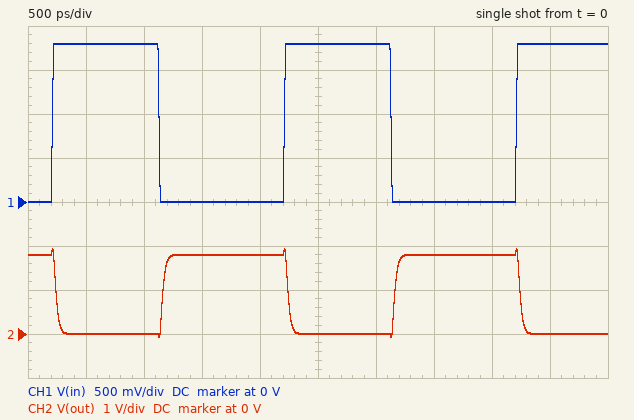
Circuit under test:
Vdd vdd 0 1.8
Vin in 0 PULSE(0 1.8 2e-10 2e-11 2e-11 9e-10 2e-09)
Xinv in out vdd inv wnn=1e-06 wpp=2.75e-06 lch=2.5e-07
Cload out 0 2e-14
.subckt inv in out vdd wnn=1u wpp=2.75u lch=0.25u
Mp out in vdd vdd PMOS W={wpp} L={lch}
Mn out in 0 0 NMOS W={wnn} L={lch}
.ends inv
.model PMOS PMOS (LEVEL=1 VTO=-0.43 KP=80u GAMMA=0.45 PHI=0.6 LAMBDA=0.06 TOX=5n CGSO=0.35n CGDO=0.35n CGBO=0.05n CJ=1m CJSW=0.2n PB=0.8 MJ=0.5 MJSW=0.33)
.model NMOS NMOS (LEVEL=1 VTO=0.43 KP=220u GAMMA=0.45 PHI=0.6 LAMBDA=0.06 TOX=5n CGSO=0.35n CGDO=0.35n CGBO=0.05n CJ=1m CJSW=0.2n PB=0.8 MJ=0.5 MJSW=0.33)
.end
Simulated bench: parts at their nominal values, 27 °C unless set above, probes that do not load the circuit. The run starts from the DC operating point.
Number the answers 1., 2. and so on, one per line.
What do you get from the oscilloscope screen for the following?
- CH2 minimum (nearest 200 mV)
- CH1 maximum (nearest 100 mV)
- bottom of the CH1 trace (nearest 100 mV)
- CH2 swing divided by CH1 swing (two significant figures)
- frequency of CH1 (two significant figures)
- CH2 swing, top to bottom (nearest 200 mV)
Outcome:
1. 0 V
2. 1.8 V
3. 0 V
4. 1.1
5. 500 MHz
6. 2.0 V
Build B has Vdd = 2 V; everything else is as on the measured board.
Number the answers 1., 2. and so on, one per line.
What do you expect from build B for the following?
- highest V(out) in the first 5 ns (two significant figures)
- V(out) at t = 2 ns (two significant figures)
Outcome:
1. 2.1 V
2. 2.0 V
